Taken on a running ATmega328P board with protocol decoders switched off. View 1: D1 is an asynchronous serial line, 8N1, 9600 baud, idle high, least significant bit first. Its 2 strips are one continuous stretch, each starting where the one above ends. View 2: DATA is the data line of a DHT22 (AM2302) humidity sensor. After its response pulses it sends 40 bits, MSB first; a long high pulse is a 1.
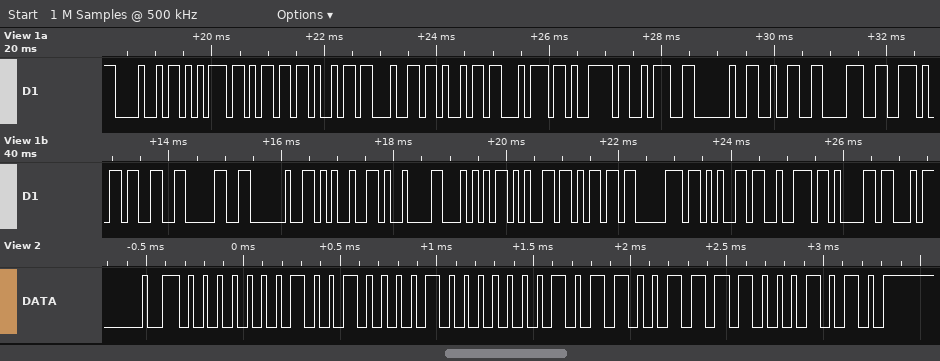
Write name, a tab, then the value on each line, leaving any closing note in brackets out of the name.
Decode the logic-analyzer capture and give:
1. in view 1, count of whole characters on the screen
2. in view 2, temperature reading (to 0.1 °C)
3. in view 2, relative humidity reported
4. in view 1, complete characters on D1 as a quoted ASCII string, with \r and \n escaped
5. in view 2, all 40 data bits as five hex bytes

in view 1, count of whole characters on the screen	25
in view 2, temperature reading	35.9 °C
in view 2, relative humidity reported	28.9 %
in view 1, complete characters on D1 as a quoted ASCII string, with \r and \n escaped	"Humidity: 28.30 %\tTempera"
in view 2, all 40 data bits as five hex bytes	01 21 01 67 8A
